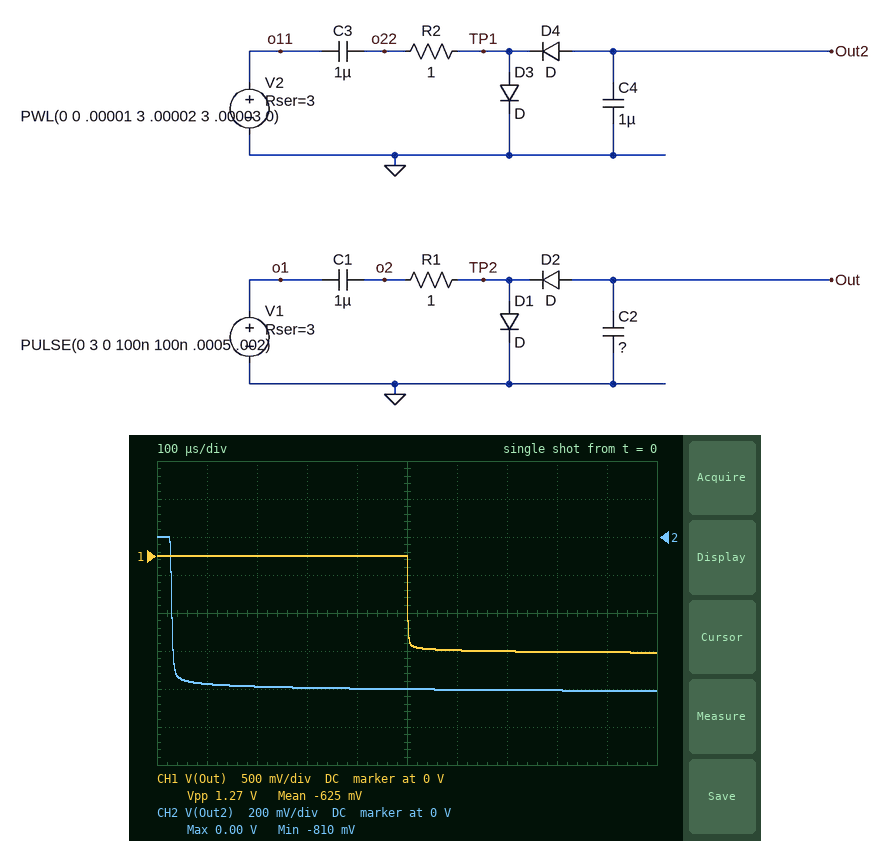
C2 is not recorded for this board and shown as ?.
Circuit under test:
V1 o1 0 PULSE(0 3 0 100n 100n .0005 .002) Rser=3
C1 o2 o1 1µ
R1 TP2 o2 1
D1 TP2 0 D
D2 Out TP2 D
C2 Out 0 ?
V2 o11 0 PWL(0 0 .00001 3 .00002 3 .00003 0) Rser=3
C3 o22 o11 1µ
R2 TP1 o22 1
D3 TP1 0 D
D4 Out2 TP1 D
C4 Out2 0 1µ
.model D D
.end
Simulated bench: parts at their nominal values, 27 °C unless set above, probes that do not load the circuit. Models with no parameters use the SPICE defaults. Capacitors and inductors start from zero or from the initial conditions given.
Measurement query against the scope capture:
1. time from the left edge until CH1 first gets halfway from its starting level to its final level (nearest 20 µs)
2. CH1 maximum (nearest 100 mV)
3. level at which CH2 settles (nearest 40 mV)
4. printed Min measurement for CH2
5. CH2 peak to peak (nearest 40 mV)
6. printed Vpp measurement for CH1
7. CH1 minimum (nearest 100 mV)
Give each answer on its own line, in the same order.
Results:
500 µs
0 V
-800 mV
-810 mV
800 mV
1.27 V
-1.3 V
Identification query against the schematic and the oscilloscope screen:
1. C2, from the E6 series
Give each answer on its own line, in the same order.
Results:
470 nF
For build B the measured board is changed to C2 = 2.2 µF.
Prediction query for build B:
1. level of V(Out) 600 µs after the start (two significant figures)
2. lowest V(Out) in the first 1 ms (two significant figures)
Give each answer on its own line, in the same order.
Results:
-560 mV
-580 mV
